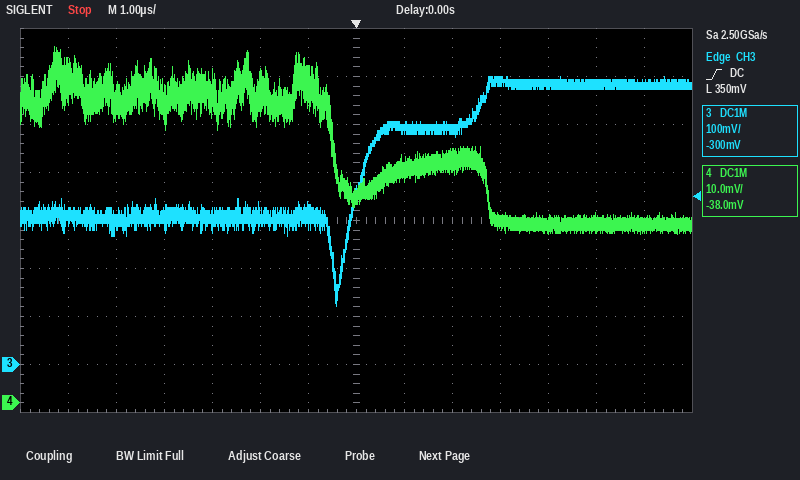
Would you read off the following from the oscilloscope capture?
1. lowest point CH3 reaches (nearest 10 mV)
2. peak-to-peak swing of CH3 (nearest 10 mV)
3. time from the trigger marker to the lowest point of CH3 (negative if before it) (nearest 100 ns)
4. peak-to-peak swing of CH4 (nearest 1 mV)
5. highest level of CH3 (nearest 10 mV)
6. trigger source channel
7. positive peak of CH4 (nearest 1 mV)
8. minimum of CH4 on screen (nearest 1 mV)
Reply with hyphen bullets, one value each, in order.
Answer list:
- 120 mV
- 480 mV
- -400 ns
- 39 mV
- 600 mV
- CH3
- 74 mV
- 35 mV
